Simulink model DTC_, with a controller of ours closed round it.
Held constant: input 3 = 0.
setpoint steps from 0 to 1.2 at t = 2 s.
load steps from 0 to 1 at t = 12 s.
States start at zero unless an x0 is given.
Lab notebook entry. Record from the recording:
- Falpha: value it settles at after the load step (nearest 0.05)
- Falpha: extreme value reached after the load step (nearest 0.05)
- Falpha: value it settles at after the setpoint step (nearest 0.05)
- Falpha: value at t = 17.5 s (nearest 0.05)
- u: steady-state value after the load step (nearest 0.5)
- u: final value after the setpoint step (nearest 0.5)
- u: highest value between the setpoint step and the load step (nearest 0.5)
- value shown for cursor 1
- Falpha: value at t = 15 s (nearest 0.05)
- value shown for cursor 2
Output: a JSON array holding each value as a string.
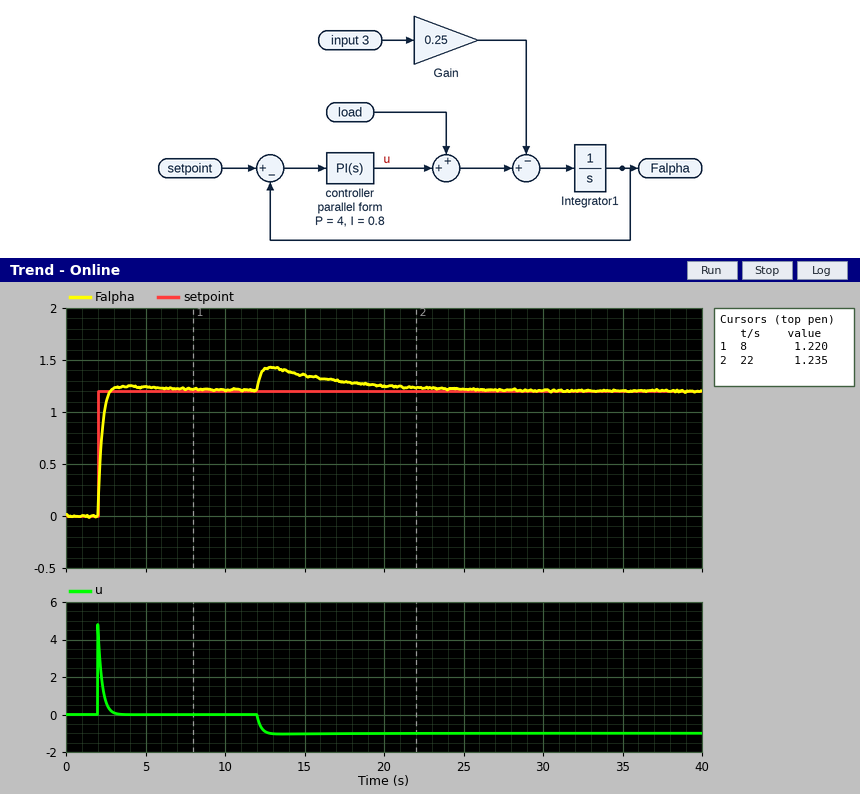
["1.20", "1.45", "1.20", "1.30", "-1.0", "0.0", "5.0", "1.220", "1.35", "1.235"]
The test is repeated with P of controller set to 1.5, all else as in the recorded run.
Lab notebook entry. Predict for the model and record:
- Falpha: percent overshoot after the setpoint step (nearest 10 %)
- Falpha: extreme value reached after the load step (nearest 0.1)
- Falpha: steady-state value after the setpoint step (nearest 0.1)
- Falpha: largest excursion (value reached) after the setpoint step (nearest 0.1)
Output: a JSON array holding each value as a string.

["20 %", "1.7", "1.2", "1.4"]
